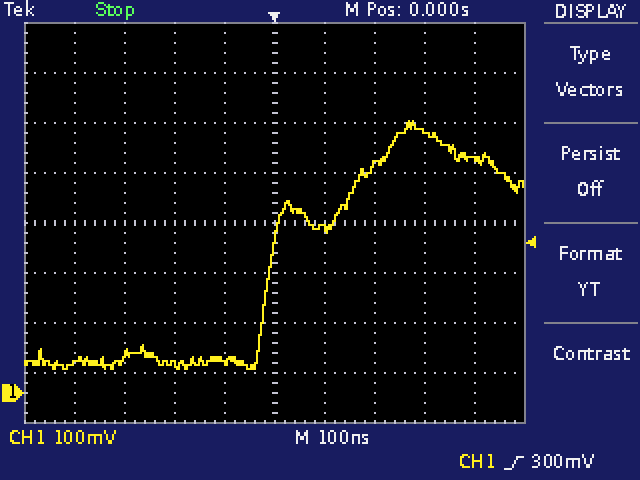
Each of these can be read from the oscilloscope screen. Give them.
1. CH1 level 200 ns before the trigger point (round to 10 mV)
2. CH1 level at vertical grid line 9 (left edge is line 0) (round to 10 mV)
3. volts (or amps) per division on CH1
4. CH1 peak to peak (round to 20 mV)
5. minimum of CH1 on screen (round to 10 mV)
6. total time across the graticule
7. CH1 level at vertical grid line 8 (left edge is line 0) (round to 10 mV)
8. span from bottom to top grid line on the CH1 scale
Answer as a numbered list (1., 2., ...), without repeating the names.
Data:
1. 60 mV
2. 470 mV
3. 100 mV
4. 500 mV
5. 50 mV
6. 1 µs
7. 520 mV
8. 800 mV
